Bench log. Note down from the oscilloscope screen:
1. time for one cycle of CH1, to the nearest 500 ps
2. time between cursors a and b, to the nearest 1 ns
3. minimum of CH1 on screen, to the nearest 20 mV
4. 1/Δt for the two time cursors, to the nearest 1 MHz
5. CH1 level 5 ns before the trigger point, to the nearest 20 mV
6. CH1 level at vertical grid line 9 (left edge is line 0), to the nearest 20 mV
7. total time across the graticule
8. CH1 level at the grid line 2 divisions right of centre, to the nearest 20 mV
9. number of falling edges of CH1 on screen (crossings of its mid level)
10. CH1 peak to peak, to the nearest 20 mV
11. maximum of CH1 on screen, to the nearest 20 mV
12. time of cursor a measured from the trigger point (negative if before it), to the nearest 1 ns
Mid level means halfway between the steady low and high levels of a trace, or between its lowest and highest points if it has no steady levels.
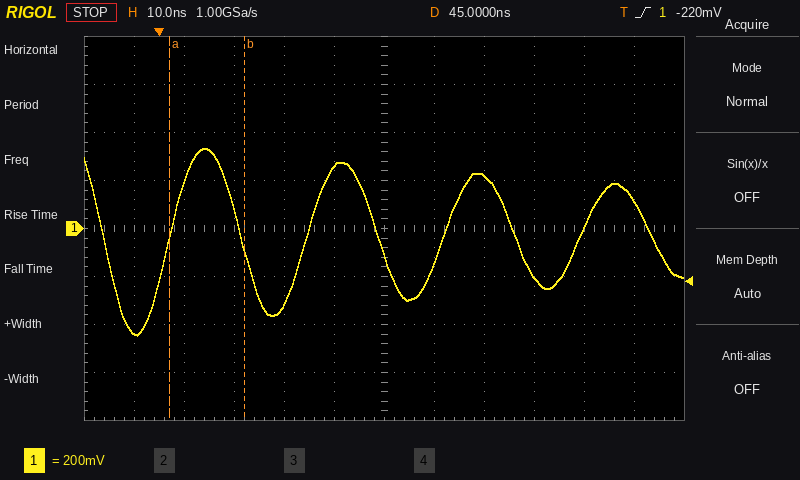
27.5 ns
15 ns
-440 mV
67 MHz
-440 mV
-200 mV
120 ns
220 mV
5
780 mV
340 mV
+2 ns
